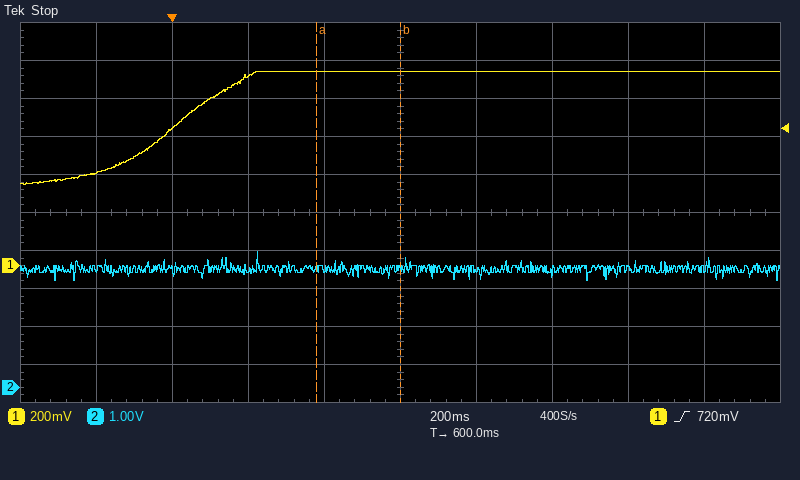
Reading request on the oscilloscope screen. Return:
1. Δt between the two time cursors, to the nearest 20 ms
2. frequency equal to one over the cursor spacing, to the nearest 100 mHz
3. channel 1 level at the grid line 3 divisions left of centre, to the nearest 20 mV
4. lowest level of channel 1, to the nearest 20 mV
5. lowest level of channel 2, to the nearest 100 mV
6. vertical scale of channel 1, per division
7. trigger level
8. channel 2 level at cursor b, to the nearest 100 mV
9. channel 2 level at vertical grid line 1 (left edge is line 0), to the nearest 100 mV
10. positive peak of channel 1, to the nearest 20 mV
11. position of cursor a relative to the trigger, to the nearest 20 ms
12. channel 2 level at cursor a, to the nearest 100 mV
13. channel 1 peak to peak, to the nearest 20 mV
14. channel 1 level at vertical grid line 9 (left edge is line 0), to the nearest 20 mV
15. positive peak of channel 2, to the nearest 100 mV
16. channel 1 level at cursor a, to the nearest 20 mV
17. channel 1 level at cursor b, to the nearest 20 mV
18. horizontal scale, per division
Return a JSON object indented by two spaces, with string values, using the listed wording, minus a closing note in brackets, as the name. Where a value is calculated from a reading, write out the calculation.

{
  "Δt between the two time cursors, to the nearest 20 ms": "220 ms",
  "frequency equal to one over the cursor spacing, to the nearest 100 mHz": "1 / 220 ms ≈ 4.5 Hz",
  "channel 1 level at the grid line 3 divisions left of centre, to the nearest 20 mV": "720 mV",
  "lowest level of channel 1, to the nearest 20 mV": "420 mV",
  "lowest level of channel 2, to the nearest 100 mV": "2.8 V",
  "vertical scale of channel 1, per division": "200 mV",
  "trigger level": "720 mV",
  "channel 2 level at cursor b, to the nearest 100 mV": "3.1 V",
  "channel 2 level at vertical grid line 1 (left edge is line 0), to the nearest 100 mV": "3.1 V",
  "positive peak of channel 1, to the nearest 20 mV": "1.02 V",
  "position of cursor a relative to the trigger, to the nearest 20 ms": "+380 ms",
  "channel 2 level at cursor a, to the nearest 100 mV": "3.1 V",
  "channel 1 peak to peak, to the nearest 20 mV": "1.02 V − (420 mV) = 600 mV",
  "channel 1 level at vertical grid line 9 (left edge is line 0), to the nearest 20 mV": "1.02 V",
  "positive peak of channel 2, to the nearest 100 mV": "3.6 V",
  "channel 1 level at cursor a, to the nearest 20 mV": "1.02 V",
  "channel 1 level at cursor b, to the nearest 20 mV": "1.02 V",
  "horizontal scale, per division": "200 ms"
}
